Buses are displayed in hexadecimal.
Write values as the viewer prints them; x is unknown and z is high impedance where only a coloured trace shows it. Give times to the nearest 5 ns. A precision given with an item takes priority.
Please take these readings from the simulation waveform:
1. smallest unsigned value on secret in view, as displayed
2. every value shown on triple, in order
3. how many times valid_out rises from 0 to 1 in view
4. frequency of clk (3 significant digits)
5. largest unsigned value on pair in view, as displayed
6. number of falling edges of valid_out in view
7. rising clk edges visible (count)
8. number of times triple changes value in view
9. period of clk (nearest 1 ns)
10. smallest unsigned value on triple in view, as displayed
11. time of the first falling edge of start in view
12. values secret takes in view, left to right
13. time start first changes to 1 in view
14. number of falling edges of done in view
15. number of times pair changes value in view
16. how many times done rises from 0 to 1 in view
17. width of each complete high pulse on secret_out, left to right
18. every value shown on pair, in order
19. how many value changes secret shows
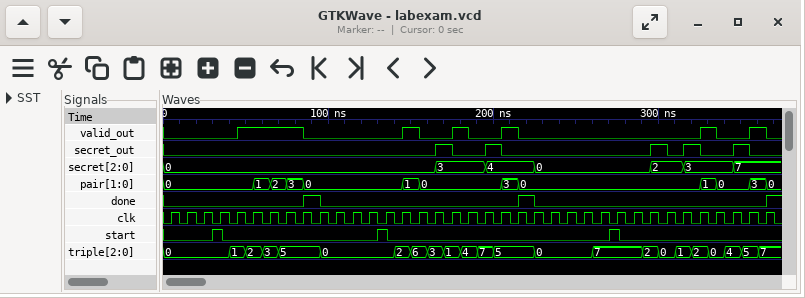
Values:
0
0, 1, 2, 3, 5, 0, 2, 6, 3, 1, 4, 7, 5, 0, 7, 2, 0, 1, 2, 0, 4, 5, 7
6
100 MHz
3
6
37
22
10 ns
0
35 ns
0, 3, 4, 0, 2, 3, 7
30 ns
2
12
3
10 ns, 10 ns, 10 ns, 10 ns, 10 ns
0, 1, 2, 3, 0, 1, 0, 3, 0, 1, 0, 3, 0
6
